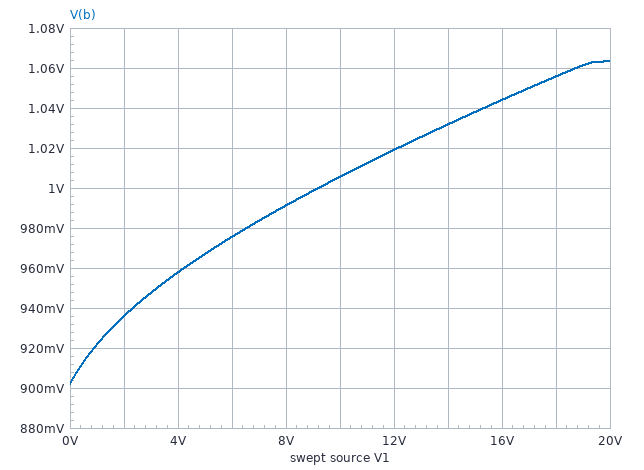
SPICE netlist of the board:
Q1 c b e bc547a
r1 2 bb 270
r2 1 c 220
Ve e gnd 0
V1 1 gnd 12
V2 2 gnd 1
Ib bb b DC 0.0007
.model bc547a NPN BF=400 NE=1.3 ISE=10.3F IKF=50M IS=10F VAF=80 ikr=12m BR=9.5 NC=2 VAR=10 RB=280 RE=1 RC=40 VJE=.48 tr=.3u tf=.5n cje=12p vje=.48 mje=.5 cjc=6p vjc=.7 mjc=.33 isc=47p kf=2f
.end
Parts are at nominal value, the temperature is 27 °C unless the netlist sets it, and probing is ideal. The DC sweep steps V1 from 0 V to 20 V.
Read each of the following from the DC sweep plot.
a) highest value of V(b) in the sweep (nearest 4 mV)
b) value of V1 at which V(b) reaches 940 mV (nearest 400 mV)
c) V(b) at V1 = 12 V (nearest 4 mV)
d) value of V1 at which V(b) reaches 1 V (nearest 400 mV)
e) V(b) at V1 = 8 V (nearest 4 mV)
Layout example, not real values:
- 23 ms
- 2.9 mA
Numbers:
- 1.064 V
- 2.4 V
- 1.020 V
- 9.2 V
- 992 mV
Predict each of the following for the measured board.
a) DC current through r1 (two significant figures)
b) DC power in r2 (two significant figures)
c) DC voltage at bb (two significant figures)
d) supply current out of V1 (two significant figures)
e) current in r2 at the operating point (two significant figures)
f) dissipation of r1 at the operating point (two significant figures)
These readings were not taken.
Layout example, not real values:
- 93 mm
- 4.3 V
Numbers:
- 700 µA
- 460 mW
- 810 mV
- 46 mA
- 46 mA
- 130 µW
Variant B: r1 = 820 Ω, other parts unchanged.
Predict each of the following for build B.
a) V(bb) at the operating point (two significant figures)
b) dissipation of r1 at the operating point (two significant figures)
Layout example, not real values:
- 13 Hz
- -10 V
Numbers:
- 430 mV
- 400 µW
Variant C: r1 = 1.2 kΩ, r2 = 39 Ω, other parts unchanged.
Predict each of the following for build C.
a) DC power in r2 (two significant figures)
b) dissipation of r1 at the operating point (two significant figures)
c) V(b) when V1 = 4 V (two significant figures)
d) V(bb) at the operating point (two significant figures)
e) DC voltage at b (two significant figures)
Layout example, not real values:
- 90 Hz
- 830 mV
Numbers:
- 240 mW
- 590 µW
- 1.0 V
- 160 mV
- 1.1 V
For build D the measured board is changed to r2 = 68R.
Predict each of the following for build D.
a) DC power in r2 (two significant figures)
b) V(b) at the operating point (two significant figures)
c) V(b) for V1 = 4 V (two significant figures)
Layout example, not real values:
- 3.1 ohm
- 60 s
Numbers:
- 400 mW
- 1.1 V
- 1.0 V
